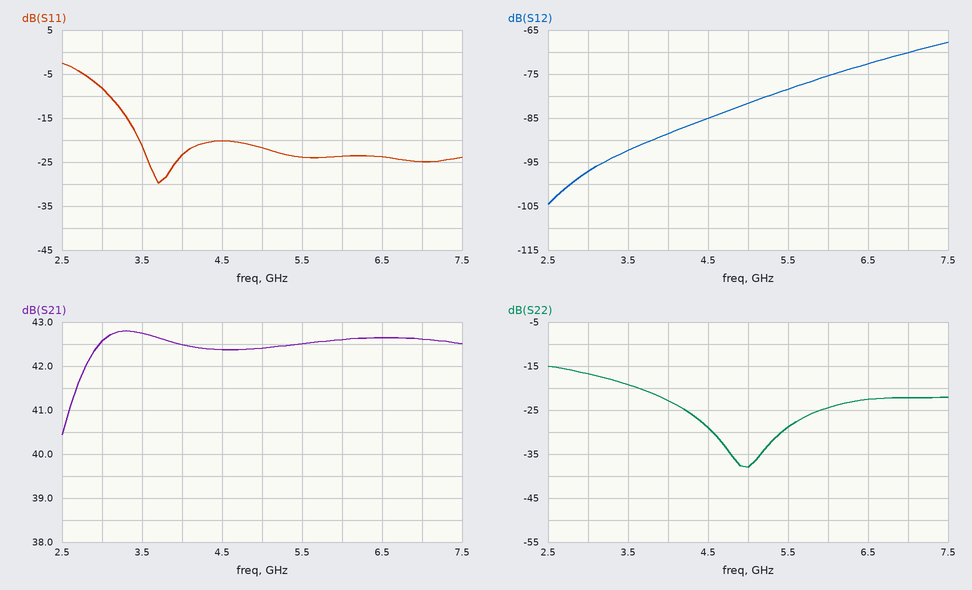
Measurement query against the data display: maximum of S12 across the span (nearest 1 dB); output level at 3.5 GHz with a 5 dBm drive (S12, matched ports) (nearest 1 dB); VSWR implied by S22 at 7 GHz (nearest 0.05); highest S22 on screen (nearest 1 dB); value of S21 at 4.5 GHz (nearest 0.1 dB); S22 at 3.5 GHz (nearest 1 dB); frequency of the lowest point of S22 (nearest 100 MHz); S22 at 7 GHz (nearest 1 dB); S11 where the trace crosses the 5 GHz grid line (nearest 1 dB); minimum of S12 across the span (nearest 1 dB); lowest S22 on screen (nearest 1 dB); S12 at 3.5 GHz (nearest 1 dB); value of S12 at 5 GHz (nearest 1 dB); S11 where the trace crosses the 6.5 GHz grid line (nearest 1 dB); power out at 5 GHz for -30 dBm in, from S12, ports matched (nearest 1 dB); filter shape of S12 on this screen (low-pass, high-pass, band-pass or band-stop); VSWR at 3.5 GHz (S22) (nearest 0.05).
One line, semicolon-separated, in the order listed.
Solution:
-68 dB; -87 dBm; 1.15; -15 dB; 42.4 dB; -19 dB; 5.0 GHz; -22 dB; -22 dB; -105 dB; -38 dB; -92 dB; -82 dB; -24 dB; -112 dBm; high-pass; 1.25
